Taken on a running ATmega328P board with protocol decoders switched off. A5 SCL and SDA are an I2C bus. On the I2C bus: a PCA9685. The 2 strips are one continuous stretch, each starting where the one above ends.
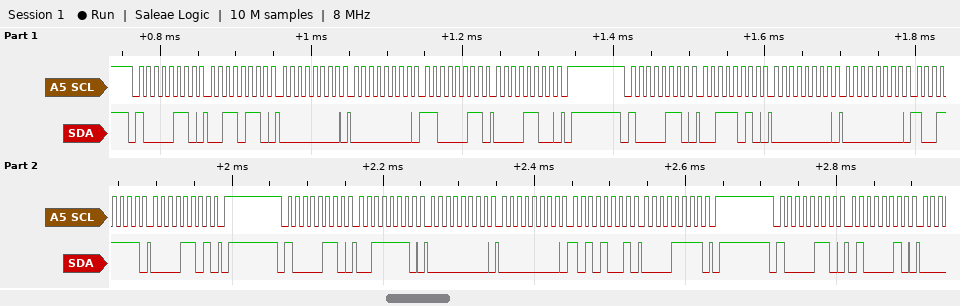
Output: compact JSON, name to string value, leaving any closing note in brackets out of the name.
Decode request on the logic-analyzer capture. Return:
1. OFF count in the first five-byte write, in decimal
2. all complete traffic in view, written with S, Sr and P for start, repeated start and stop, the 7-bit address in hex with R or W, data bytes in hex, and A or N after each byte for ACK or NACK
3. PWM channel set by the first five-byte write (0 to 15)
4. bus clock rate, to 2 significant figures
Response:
{"OFF count in the first five-byte write, in decimal": "3267", "all complete traffic in view, written with S, Sr and P for start, repeated start and stop, the 7-bit address in hex with R or W, data bytes in hex, and A or N after each byte for ACK or NACK": "S 43W A 36 A 00 A 00 A C3 A 0C A P S 43W A 3A A 00 A 00 A 9F A 0D A P S 43W A 3E A 00 A 00 A A9 A 0F A P S 43W A 42 A", "PWM channel set by the first five-byte write": "12", "bus clock rate, to 2 significant figures": "100 kHz"}
